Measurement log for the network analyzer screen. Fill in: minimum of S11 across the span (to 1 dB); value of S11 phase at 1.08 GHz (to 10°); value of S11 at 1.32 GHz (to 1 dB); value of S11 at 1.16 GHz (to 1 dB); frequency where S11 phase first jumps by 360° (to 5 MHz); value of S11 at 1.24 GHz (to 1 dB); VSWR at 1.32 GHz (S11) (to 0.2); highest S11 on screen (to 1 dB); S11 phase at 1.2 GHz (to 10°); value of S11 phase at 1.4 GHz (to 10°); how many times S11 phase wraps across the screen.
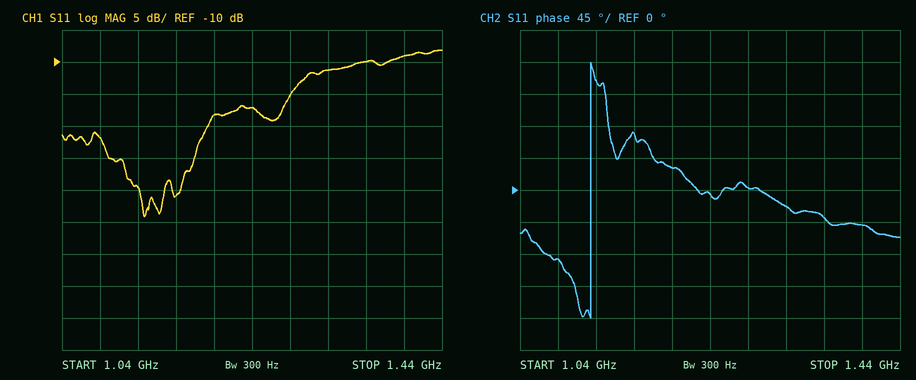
-34 dB
-100°
-11 dB
-31 dB
1.115 GHz
-17 dB
1.8
-8 dB
30°
-50°
1
